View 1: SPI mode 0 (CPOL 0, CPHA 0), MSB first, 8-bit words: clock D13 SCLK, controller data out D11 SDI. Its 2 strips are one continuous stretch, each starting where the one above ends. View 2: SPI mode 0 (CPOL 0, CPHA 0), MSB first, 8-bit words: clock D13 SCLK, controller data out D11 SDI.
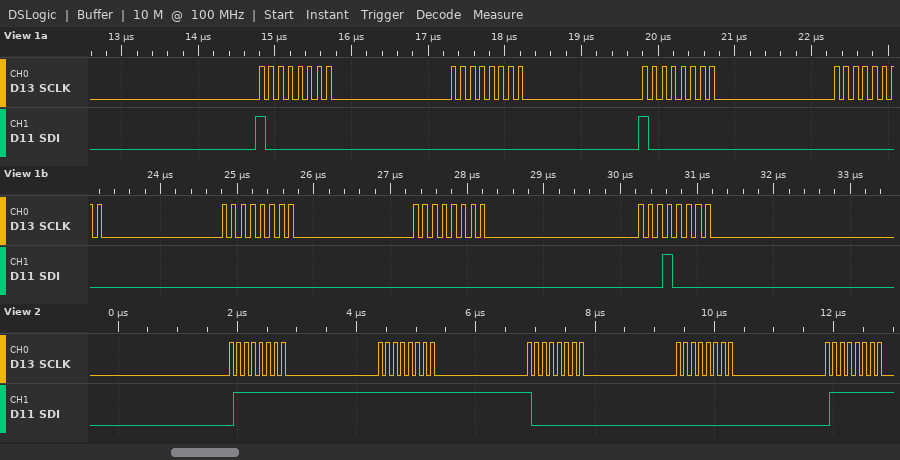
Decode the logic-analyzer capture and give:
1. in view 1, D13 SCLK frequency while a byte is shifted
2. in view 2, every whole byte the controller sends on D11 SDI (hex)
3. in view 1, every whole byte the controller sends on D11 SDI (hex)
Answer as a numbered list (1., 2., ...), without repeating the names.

1. 8 MHz
2. 0x7F 0xFF 0x80 0x00 0x7F
3. 80 00 80 00 00 00 10
